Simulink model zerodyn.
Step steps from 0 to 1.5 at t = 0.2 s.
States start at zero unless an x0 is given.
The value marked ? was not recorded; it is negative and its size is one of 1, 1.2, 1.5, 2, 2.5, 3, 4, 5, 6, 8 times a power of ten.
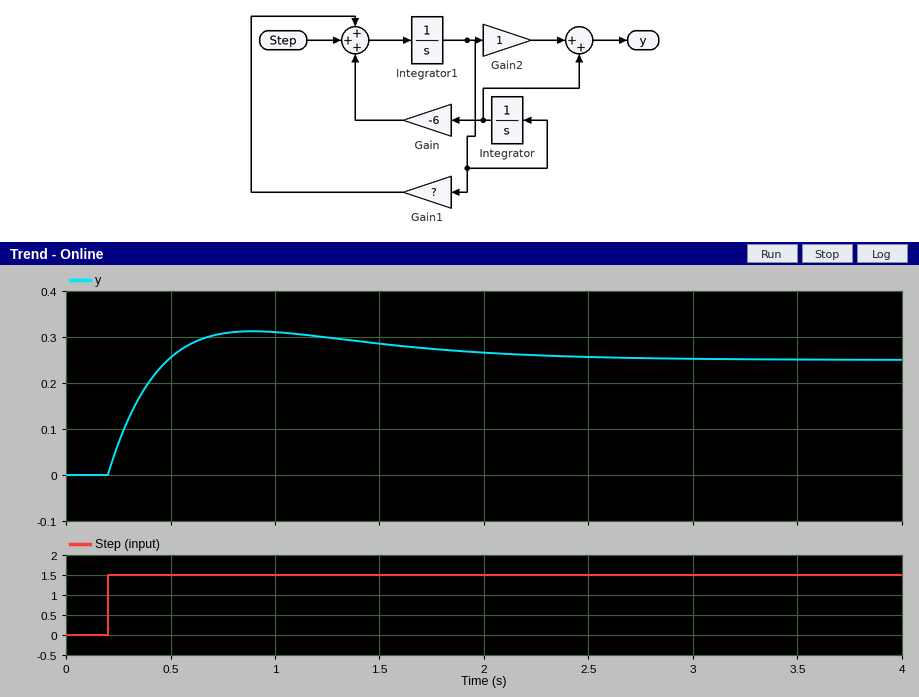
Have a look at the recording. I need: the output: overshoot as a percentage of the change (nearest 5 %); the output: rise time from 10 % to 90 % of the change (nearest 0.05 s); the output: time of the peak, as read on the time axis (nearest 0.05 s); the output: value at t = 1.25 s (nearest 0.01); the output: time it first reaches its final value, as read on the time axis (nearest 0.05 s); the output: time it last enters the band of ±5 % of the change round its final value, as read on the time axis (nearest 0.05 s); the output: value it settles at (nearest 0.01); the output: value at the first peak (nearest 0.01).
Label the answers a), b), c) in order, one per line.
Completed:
a) 25 %
b) 0.20 s
c) 0.90 s
d) 0.30
e) 0.50 s
f) 2.15 s
g) 0.25
h) 0.31
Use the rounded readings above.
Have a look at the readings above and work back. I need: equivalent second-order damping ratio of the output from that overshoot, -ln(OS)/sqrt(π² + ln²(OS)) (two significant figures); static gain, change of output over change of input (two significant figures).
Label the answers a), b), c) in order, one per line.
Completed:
a) 0.40
b) 0.17
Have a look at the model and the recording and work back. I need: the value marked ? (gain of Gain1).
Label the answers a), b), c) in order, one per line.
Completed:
a) -5
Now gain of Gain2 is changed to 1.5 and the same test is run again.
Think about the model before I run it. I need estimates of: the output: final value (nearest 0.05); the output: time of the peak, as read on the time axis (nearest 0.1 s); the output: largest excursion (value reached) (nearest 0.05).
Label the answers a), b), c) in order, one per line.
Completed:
a) 0.25
b) 0.8 s
c) 0.40
